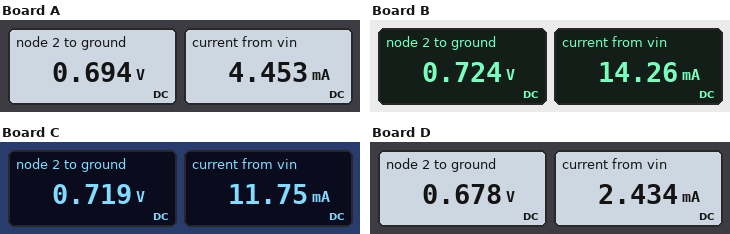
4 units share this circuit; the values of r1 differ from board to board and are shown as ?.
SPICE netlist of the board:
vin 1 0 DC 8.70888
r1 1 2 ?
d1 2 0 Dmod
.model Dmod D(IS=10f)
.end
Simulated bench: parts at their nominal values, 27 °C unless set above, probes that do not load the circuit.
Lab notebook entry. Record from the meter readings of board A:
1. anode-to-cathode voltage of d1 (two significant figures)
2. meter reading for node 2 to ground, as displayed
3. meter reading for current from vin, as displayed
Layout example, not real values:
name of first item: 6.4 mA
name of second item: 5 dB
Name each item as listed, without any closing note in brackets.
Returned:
anode-to-cathode voltage of d1: 690 mV
meter reading for node 2 to ground, as displayed: 0.694 V
meter reading for current from vin, as displayed: 4.453 mA
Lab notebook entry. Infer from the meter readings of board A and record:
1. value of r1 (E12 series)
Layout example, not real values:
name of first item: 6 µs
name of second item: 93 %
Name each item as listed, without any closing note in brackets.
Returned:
value of r1: 1.8 kΩ
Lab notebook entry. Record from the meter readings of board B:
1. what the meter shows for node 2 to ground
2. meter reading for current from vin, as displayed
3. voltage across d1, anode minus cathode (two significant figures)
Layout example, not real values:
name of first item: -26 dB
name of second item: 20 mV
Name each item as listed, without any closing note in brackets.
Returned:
what the meter shows for node 2 to ground: 0.724 V
meter reading for current from vin, as displayed: 14.26 mA
voltage across d1, anode minus cathode: 720 mV
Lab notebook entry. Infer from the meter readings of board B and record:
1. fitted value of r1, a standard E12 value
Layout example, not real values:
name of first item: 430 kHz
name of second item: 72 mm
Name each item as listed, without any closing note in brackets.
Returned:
fitted value of r1, a standard E12 value: 560 Ω
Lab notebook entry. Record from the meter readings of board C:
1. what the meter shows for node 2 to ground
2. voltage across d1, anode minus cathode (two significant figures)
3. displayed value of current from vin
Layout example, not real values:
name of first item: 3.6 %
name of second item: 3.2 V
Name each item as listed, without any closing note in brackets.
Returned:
what the meter shows for node 2 to ground: 0.719 V
voltage across d1, anode minus cathode: 720 mV
displayed value of current from vin: 11.75 mA
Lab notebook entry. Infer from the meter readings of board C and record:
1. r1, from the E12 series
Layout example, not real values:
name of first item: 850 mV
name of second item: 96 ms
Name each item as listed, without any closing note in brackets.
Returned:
r1, from the E12 series: 680 Ω
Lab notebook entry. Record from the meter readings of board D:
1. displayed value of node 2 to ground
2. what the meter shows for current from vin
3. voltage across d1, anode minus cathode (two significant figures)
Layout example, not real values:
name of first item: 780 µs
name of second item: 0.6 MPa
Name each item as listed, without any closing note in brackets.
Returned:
displayed value of node 2 to ground: 0.678 V
what the meter shows for current from vin: 2.434 mA
voltage across d1, anode minus cathode: 680 mV
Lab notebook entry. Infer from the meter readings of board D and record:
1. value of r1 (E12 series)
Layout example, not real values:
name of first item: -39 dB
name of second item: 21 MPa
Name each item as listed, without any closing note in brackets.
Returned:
value of r1: 3.3 kΩ
